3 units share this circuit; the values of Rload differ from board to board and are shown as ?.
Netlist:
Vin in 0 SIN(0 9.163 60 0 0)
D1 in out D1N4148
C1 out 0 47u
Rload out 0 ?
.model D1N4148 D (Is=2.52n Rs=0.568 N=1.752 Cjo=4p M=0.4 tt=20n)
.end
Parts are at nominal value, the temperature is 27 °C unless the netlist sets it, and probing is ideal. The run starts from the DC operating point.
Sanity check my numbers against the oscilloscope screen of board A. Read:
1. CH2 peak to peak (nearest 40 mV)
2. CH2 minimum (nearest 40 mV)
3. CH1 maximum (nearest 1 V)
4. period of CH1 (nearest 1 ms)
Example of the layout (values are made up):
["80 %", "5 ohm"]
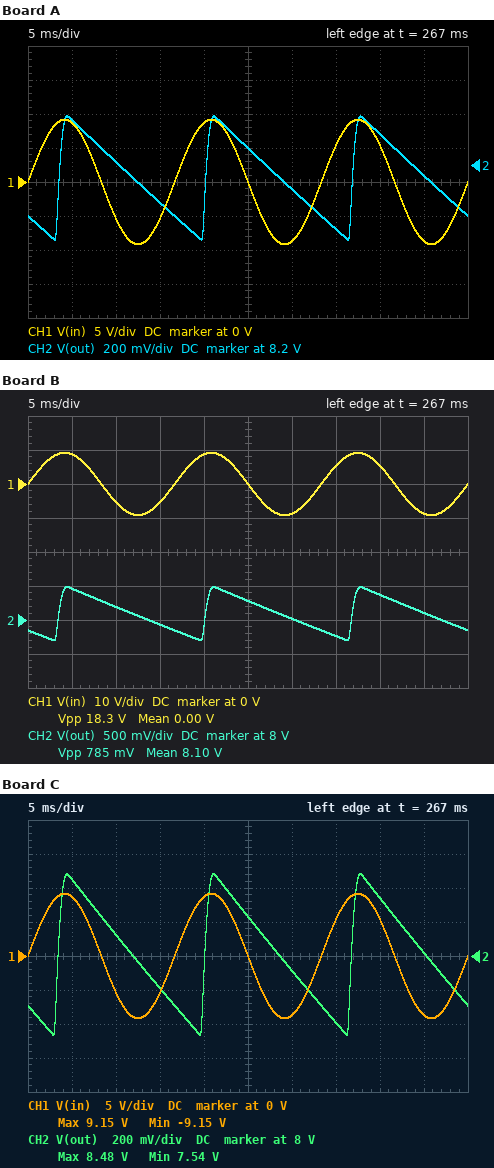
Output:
["720 mV", "7.76 V", "9 V", "17 ms"]
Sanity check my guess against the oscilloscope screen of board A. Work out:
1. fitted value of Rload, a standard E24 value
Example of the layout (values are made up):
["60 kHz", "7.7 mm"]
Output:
["3.6 kΩ"]
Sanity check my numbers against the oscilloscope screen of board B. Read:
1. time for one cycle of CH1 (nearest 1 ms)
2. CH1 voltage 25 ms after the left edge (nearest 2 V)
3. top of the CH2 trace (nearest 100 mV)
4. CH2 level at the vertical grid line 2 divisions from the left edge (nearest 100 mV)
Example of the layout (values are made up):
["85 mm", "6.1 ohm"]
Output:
["17 ms", "0 V", "8.5 V", "8.2 V"]
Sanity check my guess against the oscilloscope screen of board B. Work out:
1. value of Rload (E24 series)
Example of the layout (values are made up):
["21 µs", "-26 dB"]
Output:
["3.3 kΩ"]
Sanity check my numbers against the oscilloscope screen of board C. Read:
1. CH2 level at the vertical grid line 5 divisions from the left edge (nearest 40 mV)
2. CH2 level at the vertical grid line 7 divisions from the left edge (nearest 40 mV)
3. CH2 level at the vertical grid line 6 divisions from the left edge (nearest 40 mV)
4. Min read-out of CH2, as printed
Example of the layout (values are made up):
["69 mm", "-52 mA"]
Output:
["8.24 V", "7.60 V", "7.92 V", "7.54 V"]
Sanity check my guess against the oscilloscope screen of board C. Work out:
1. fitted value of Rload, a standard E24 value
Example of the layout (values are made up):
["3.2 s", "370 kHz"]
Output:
["2.7 kΩ"]
